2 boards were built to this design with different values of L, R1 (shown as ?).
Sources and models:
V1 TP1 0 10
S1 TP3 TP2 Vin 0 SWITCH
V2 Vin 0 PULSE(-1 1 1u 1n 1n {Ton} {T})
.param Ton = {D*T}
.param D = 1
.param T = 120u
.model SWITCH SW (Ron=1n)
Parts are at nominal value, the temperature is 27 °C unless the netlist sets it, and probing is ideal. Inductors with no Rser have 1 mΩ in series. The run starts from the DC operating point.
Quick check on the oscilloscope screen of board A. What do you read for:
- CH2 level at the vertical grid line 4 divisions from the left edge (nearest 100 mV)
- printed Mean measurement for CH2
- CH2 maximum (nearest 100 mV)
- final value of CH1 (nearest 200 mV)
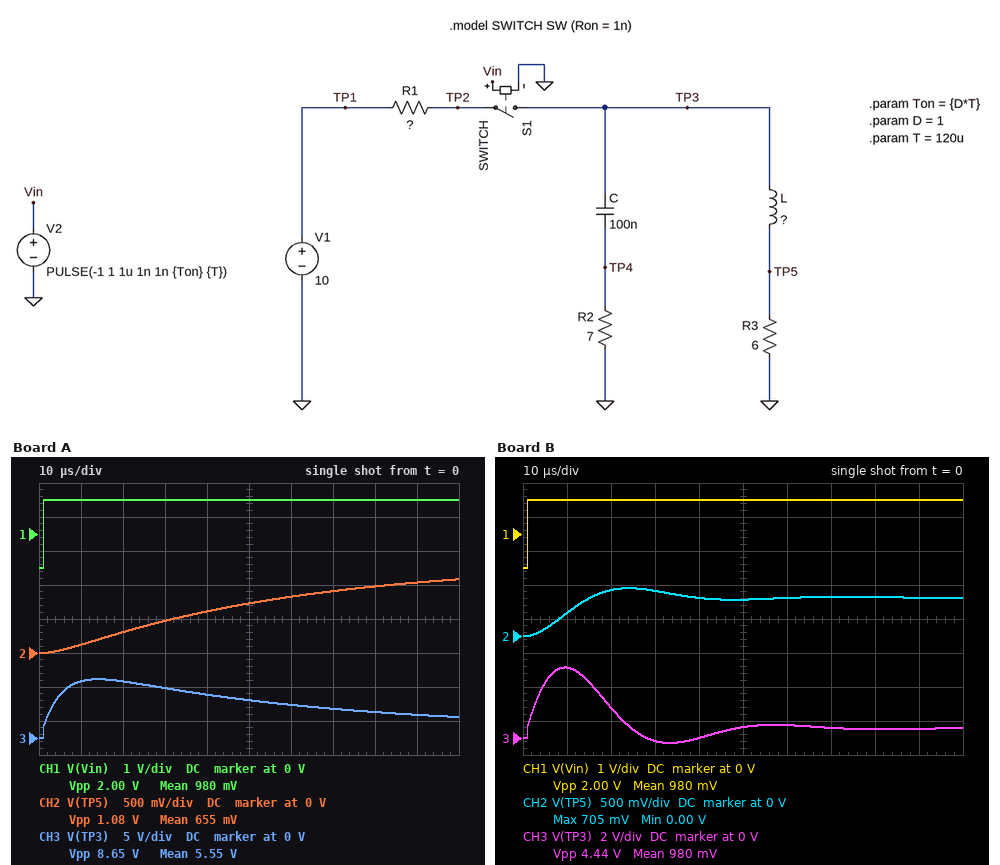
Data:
600 mV
655 mV
1.1 V
1.0 V
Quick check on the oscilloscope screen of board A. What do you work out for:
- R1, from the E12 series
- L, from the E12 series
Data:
39 Ω
2.7 mH
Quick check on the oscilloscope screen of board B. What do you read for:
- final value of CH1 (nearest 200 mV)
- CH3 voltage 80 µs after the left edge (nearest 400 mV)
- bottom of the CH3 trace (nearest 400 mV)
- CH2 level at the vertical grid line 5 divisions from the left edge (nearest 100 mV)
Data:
1.0 V
400 mV
-400 mV
500 mV
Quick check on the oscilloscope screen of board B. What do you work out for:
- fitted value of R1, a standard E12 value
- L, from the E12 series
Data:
100 Ω
470 µH
